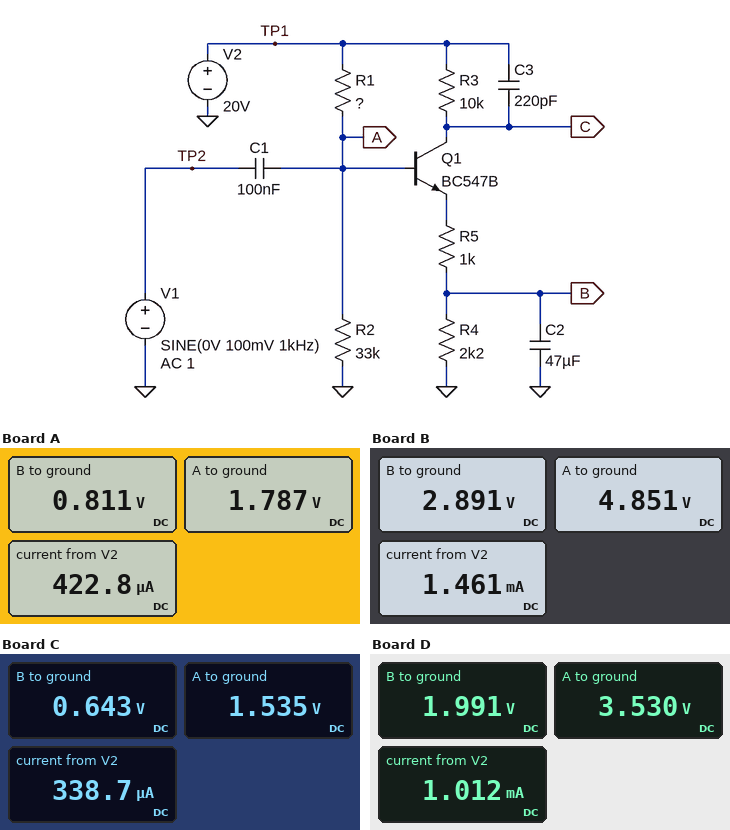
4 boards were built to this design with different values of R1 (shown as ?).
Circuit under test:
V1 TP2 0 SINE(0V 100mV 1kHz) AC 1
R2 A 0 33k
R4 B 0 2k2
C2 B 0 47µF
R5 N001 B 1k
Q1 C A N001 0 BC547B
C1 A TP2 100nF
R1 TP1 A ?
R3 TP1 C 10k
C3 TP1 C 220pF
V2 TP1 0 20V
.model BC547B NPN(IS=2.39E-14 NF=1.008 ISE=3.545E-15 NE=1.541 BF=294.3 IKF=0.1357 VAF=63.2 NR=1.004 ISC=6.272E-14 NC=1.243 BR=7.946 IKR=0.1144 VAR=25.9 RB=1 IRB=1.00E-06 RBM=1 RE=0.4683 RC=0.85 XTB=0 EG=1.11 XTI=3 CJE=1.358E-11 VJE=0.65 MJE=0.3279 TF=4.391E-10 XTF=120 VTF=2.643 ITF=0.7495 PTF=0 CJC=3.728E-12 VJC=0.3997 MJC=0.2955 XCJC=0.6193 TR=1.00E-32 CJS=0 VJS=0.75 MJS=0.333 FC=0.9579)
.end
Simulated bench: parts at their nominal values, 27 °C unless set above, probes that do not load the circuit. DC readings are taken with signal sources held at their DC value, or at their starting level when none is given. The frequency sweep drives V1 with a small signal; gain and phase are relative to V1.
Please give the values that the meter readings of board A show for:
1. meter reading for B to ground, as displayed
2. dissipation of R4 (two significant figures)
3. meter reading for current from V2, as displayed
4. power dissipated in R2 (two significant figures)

0.811 V
300 µW
422.8 µA
97 µW
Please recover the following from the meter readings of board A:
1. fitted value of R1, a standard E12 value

330 kΩ
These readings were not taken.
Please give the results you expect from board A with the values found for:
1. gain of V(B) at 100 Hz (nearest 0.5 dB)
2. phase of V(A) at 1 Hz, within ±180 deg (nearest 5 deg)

-31.5 dB
90 deg
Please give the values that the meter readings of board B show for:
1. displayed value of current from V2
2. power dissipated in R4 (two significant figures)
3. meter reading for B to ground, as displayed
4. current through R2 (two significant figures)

1.461 mA
3.8 mW
2.891 V
150 µA
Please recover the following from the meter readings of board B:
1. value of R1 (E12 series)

100 kΩ
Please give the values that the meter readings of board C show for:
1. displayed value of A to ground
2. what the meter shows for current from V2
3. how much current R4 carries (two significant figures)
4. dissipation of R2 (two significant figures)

1.535 V
338.7 µA
290 µA
71 µW
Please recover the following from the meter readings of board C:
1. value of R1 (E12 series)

390 kΩ
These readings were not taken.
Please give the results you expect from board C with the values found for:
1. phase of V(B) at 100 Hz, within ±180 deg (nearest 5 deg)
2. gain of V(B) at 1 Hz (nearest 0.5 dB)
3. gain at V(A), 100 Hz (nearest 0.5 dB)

-60 deg
-38.5 dB
-1.0 dB
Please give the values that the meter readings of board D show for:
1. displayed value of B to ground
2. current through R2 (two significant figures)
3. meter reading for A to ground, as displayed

1.991 V
110 µA
3.530 V
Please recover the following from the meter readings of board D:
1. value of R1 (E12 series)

150 kΩ
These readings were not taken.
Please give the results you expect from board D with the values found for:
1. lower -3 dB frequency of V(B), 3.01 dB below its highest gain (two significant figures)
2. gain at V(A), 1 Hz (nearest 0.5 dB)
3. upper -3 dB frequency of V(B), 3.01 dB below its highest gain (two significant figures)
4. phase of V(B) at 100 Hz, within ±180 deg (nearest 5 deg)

4.0 Hz
-35.5 dB
73 Hz
-55 deg
